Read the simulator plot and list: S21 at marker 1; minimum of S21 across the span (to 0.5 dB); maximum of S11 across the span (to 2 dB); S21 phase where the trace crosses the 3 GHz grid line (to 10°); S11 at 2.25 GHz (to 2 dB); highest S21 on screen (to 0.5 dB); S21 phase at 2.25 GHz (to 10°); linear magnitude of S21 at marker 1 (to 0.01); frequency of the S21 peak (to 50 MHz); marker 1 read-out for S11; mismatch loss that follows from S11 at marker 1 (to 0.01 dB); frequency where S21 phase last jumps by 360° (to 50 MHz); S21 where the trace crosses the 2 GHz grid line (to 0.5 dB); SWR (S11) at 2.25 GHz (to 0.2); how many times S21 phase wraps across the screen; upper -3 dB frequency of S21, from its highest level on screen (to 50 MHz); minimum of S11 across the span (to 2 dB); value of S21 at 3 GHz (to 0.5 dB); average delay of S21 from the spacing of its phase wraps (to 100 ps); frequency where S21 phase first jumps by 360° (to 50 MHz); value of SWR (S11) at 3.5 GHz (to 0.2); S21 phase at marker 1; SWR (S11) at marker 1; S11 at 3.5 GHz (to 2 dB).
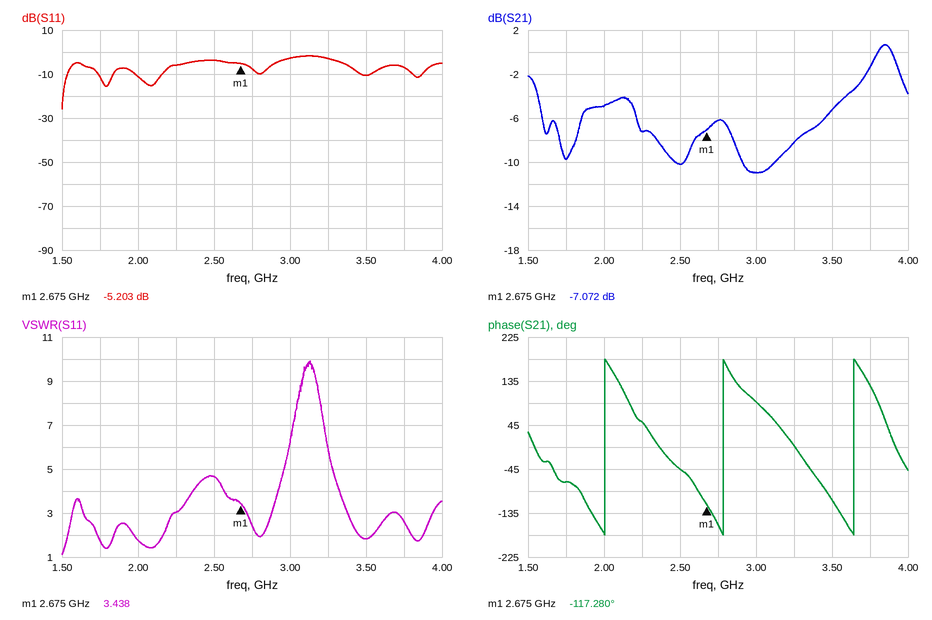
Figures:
-7.072 dB
-11.0 dB
-2 dB
90°
-6 dB
0.5 dB
50°
0.44
3.85 GHz
-5.203 dB
1.56 dB
3.65 GHz
-5.0 dB
3.0
3
3.95 GHz
-26 dB
-11.0 dB
1.2 ns
2.00 GHz
1.8
-117.280°
3.438
-10 dB
